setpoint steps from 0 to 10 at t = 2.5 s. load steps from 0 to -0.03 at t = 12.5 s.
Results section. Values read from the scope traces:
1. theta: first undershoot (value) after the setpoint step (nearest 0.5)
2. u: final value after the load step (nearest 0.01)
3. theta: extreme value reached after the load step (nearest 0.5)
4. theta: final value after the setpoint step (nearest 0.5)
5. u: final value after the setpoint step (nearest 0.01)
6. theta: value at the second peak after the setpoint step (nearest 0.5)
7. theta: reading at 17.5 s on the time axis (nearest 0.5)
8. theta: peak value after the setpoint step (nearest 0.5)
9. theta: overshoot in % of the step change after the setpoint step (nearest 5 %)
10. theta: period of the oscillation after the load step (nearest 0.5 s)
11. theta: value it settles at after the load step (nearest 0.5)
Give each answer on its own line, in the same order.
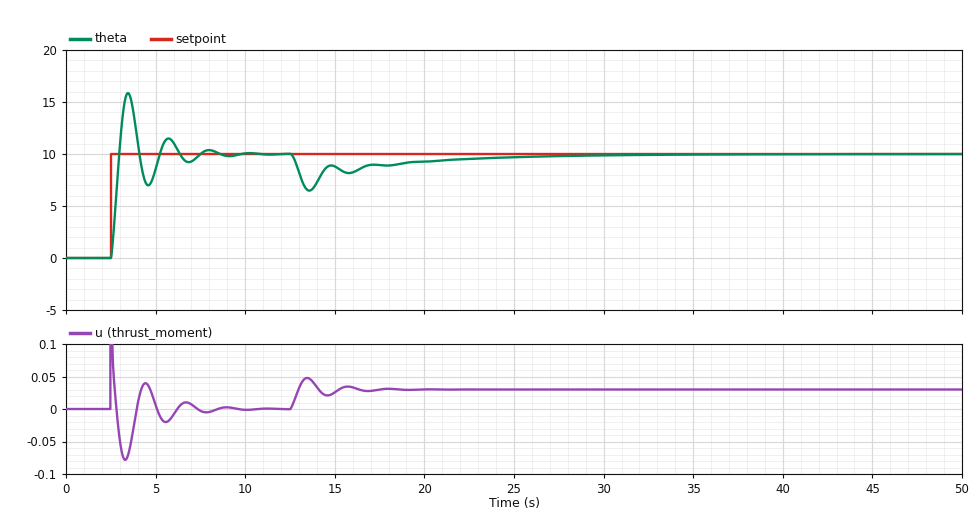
7.0
0.03
6.5
10.0
0.00
11.5
9.0
16.0
60 %
2.0 s
10.0
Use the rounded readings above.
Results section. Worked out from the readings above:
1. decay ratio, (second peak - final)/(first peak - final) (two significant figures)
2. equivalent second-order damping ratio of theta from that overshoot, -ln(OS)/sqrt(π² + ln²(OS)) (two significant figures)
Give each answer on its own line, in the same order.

0.25
0.16
